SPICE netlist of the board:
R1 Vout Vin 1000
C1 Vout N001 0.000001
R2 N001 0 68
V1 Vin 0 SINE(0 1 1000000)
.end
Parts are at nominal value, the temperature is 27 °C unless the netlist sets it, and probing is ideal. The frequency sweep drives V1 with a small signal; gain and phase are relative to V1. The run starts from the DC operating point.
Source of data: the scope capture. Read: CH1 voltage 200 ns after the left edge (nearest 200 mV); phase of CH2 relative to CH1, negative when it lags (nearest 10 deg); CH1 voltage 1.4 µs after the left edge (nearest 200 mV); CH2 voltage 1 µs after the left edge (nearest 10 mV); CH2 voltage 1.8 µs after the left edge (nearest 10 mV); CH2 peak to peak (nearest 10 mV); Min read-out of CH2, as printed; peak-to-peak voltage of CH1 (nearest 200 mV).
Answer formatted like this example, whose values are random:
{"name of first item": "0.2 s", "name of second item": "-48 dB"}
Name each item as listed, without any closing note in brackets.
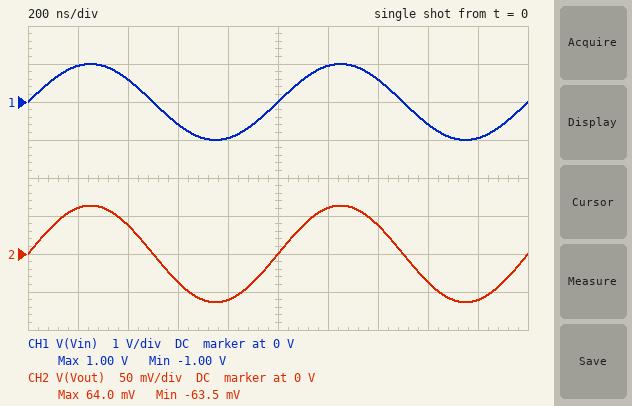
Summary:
{"CH1 voltage 200 ns after the left edge": "1.0 V", "phase of CH2 relative to CH1, negative when it lags": "0 deg", "CH1 voltage 1.4 µs after the left edge": "600 mV", "CH2 voltage 1 µs after the left edge": "0 V", "CH2 voltage 1.8 µs after the left edge": "-60 mV", "CH2 peak to peak": "130 mV", "Min read-out of CH2, as printed": "-63.5 mV", "peak-to-peak voltage of CH1": "2.0 V"}
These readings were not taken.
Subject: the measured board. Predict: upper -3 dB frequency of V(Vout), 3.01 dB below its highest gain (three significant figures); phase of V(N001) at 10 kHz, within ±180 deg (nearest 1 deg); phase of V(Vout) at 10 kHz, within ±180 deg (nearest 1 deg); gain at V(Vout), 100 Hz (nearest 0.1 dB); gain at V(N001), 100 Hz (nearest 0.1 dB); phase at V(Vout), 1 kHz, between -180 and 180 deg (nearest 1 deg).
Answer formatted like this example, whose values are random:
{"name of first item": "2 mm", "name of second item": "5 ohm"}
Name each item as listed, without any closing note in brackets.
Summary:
{"upper -3 dB frequency of V(Vout), 3.01 dB below its highest gain": "150 Hz", "phase of V(N001) at 10 kHz, within ±180 deg": "1 deg", "phase of V(Vout) at 10 kHz, within ±180 deg": "-12 deg", "gain at V(Vout), 100 Hz": "-1.6 dB", "gain at V(N001), 100 Hz": "-29.0 dB", "phase at V(Vout), 1 kHz, between -180 and 180 deg": "-58 deg"}
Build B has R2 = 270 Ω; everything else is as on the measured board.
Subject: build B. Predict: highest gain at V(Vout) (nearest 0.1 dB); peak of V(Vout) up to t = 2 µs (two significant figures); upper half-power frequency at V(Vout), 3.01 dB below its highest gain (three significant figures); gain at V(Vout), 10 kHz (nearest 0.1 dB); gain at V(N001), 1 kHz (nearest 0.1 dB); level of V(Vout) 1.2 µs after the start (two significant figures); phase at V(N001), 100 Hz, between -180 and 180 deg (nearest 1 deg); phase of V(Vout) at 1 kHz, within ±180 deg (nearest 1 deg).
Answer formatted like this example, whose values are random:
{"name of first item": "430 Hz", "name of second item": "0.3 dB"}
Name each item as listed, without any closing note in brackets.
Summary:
{"highest gain at V(Vout)": "0 dB", "peak of V(Vout) up to t = 2 µs": "210 mV", "upper half-power frequency at V(Vout), 3.01 dB below its highest gain": "131 Hz", "gain at V(Vout), 10 kHz": "-13.4 dB", "gain at V(N001), 1 kHz": "-13.5 dB", "level of V(Vout) 1.2 µs after the start": "200 mV", "phase at V(N001), 100 Hz, between -180 and 180 deg": "51 deg", "phase of V(Vout) at 1 kHz, within ±180 deg": "-23 deg"}
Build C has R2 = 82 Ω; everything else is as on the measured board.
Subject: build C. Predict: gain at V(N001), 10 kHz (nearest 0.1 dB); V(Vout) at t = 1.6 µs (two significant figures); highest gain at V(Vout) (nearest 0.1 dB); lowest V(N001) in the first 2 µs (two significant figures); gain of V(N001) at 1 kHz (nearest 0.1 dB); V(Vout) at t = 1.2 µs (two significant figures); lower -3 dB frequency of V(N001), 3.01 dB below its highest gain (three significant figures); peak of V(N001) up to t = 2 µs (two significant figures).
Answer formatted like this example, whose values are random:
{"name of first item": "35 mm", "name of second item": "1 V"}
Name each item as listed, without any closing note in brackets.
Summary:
{"gain at V(N001), 10 kHz": "-22.4 dB", "V(Vout) at t = 1.6 µs": "-44 mV", "highest gain at V(Vout)": "0 dB", "lowest V(N001) in the first 2 µs": "-76 mV", "gain of V(N001) at 1 kHz": "-22.5 dB", "V(Vout) at t = 1.2 µs": "72 mV", "lower -3 dB frequency of V(N001), 3.01 dB below its highest gain": "147 Hz", "peak of V(N001) up to t = 2 µs": "76 mV"}
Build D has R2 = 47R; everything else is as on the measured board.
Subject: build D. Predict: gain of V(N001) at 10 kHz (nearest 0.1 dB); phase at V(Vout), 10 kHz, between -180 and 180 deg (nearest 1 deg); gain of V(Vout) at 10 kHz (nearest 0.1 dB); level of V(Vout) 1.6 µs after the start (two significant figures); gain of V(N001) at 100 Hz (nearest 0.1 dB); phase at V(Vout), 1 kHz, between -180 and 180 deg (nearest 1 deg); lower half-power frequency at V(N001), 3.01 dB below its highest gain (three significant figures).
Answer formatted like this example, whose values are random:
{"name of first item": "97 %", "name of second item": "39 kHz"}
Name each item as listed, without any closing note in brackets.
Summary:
{"gain of V(N001) at 10 kHz": "-27.0 dB", "phase at V(Vout), 10 kHz, between -180 and 180 deg": "-18 deg", "gain of V(Vout) at 10 kHz": "-26.5 dB", "level of V(Vout) 1.6 µs after the start": "-26 mV", "gain of V(N001) at 100 Hz": "-32.2 dB", "phase at V(Vout), 1 kHz, between -180 and 180 deg": "-65 deg", "lower half-power frequency at V(N001), 3.01 dB below its highest gain": "152 Hz"}
